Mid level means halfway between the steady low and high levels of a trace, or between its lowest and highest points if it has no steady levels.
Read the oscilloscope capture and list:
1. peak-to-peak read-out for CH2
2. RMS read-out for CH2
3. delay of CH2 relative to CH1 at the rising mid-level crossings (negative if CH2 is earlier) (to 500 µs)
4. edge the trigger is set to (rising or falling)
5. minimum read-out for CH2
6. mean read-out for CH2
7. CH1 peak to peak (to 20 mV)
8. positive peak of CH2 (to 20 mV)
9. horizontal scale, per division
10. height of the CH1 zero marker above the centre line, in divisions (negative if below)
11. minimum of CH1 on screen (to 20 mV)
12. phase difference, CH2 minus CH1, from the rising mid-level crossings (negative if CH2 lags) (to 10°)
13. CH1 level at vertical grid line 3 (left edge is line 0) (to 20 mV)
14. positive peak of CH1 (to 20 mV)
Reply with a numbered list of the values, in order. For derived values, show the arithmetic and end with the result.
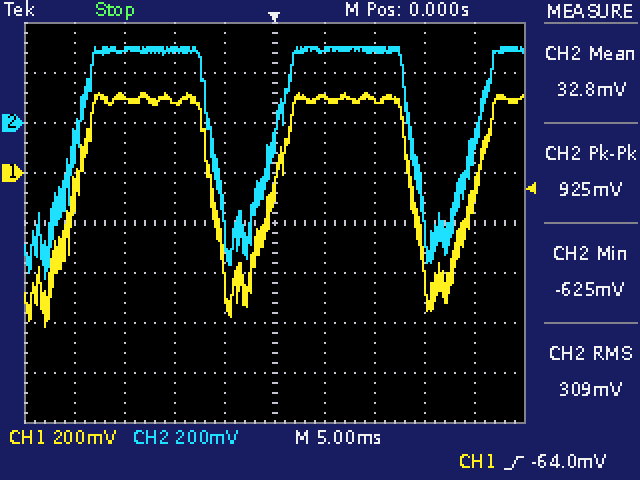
1. 925 mV
2. 309 mV
3. 0.0 ms
4. rising
5. -625 mV
6. 32.8 mV
7. 320 mV − (-620 mV) = 940 mV
8. 300 mV
9. 5 ms
10. +1.0 div
11. -620 mV
12. 0°
13. 280 mV
14. 320 mV
